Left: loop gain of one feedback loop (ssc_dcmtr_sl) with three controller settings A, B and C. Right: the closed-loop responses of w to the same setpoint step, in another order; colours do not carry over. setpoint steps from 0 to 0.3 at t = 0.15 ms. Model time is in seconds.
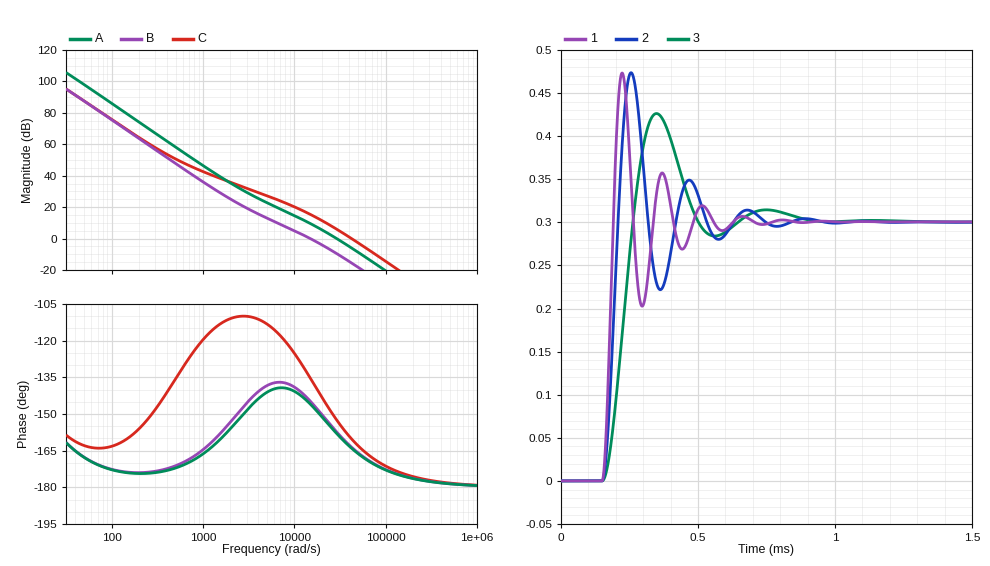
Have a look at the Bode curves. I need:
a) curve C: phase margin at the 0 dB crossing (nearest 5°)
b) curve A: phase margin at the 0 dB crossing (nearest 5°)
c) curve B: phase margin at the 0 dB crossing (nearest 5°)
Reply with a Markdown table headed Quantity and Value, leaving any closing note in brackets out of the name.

| Quantity | Value |
|---|---|
| curve C: phase margin at the 0 dB crossing | 20° |
| curve A: phase margin at the 0 dB crossing | 20° |
| curve B: phase margin at the 0 dB crossing | 35° |
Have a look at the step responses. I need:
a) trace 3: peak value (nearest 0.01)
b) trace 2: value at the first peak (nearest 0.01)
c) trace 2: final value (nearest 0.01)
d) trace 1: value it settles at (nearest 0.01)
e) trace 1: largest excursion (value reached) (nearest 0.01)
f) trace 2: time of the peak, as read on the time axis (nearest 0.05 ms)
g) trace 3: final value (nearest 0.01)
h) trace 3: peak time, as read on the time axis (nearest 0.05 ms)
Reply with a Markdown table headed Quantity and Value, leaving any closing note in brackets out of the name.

| Quantity | Value |
|---|---|
| trace 3: peak value | 0.43 |
| trace 2: value at the first peak | 0.47 |
| trace 2: final value | 0.30 |
| trace 1: value it settles at | 0.30 |
| trace 1: largest excursion (value reached) | 0.47 |
| trace 2: time of the peak, as read on the time axis | 0.25 ms |
| trace 3: final value | 0.30 |
| trace 3: peak time, as read on the time axis | 0.35 ms |
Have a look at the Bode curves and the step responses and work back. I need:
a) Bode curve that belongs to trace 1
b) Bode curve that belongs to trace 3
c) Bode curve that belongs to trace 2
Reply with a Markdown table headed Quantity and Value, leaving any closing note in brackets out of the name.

| Quantity | Value |
|---|---|
| Bode curve that belongs to trace 1 | C |
| Bode curve that belongs to trace 3 | B |
| Bode curve that belongs to trace 2 | A |
